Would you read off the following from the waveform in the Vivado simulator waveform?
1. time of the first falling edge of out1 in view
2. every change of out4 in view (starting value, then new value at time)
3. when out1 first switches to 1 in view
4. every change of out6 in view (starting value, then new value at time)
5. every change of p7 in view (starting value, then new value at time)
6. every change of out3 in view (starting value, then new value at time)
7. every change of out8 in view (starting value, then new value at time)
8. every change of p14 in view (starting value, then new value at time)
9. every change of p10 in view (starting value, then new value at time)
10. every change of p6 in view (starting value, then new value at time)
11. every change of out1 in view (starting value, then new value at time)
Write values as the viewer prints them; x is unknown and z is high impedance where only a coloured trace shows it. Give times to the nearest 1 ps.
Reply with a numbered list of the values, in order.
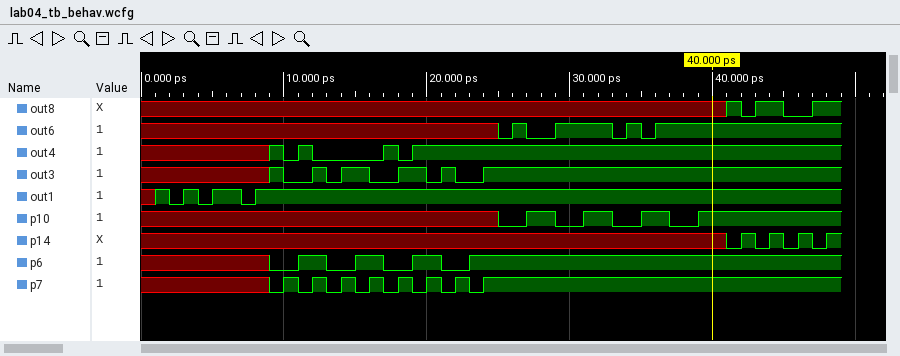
1. 2 ps
2. x, 1 at 9 ps, 0 at 10 ps, 1 at 11 ps, 0 at 12 ps, 1 at 17 ps, 0 at 18 ps, 1 at 19 ps
3. 1 ps
4. x, 0 at 25 ps, 1 at 26 ps, 0 at 27 ps, 1 at 29 ps, 0 at 33 ps, 1 at 34 ps, 0 at 35 ps, 1 at 36 ps
5. x, 0 at 9 ps, 1 at 10 ps, 0 at 11 ps, 1 at 12 ps, 0 at 13 ps, 1 at 14 ps, 0 at 15 ps, 1 at 16 ps, 0 at 17 ps, 1 at 18 ps, 0 at 19 ps, 1 at 20 ps, 0 at 21 ps, 1 at 22 ps, 0 at 23 ps, 1 at 24 ps
6. x, 1 at 9 ps, 0 at 10 ps, 1 at 12 ps, 0 at 13 ps, 1 at 14 ps, 0 at 16 ps, 1 at 18 ps, 0 at 20 ps, 1 at 21 ps, 0 at 22 ps, 1 at 24 ps
7. x, 1 at 41 ps, 0 at 42 ps, 1 at 43 ps, 0 at 45 ps, 1 at 47 ps
8. x, 0 at 41 ps, 1 at 42 ps, 0 at 43 ps, 1 at 44 ps, 0 at 45 ps, 1 at 46 ps, 0 at 47 ps, 1 at 48 ps
9. x, 0 at 25 ps, 1 at 27 ps, 0 at 29 ps, 1 at 31 ps, 0 at 33 ps, 1 at 35 ps, 0 at 37 ps, 1 at 39 ps
10. x, 0 at 9 ps, 1 at 11 ps, 0 at 13 ps, 1 at 15 ps, 0 at 17 ps, 1 at 19 ps, 0 at 21 ps, 1 at 23 ps
11. x, 1 at 1 ps, 0 at 2 ps, 1 at 3 ps, 0 at 4 ps, 1 at 5 ps, 0 at 7 ps, 1 at 8 ps
